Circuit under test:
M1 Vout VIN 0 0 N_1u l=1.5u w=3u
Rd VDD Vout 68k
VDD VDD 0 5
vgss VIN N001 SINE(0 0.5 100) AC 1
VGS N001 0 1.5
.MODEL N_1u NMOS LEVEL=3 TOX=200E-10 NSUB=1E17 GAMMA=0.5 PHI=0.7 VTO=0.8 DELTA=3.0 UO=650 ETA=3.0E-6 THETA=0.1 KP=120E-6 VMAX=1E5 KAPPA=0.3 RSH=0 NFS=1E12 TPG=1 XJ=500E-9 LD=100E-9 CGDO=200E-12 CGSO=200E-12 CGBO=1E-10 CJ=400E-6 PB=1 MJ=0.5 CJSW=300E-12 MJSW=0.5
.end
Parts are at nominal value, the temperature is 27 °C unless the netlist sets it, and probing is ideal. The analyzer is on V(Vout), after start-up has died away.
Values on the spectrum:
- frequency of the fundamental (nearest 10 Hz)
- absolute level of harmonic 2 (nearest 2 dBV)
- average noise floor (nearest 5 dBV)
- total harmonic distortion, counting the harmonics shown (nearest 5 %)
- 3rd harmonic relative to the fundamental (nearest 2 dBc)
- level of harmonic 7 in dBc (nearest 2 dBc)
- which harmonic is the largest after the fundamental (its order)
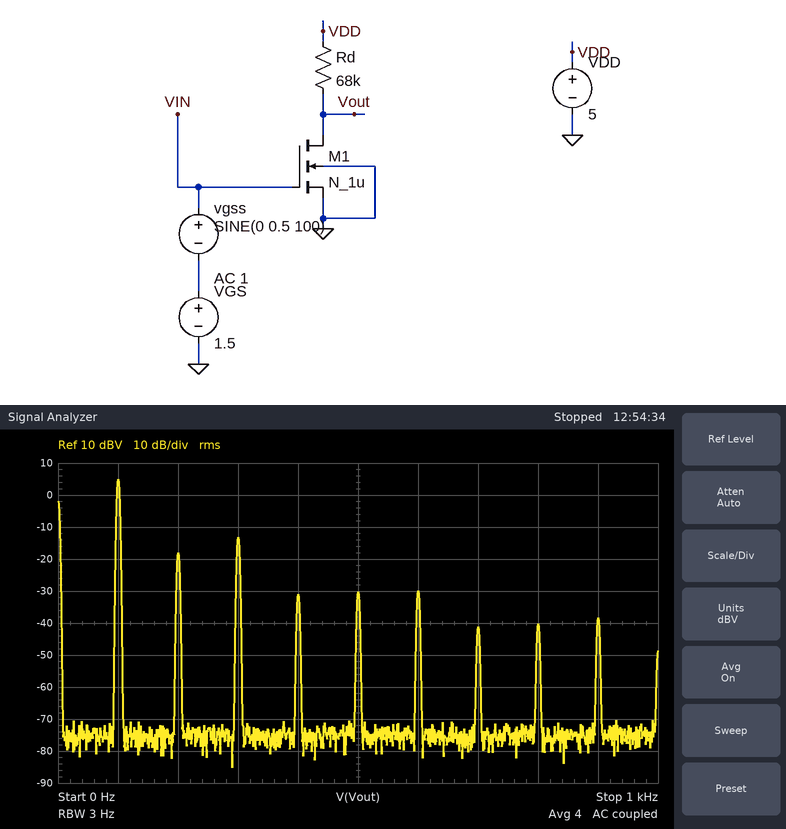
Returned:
100 Hz
-18 dBV
-75 dBV
15 %
-18 dBc
-46 dBc
3
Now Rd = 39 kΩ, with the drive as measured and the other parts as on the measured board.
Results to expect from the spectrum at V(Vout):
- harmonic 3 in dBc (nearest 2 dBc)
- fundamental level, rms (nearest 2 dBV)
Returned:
-34 dBc
2 dBV
